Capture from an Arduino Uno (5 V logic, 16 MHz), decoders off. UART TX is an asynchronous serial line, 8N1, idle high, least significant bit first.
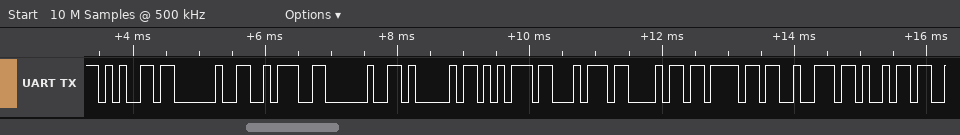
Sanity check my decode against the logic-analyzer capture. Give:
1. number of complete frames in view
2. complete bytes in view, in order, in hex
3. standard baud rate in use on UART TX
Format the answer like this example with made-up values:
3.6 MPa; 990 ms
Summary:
11; 0x65 0x20 0x3A 0x20 0x41 0x75 0x74 0x68 0x6F 0x72 0x69; 9600 baud
